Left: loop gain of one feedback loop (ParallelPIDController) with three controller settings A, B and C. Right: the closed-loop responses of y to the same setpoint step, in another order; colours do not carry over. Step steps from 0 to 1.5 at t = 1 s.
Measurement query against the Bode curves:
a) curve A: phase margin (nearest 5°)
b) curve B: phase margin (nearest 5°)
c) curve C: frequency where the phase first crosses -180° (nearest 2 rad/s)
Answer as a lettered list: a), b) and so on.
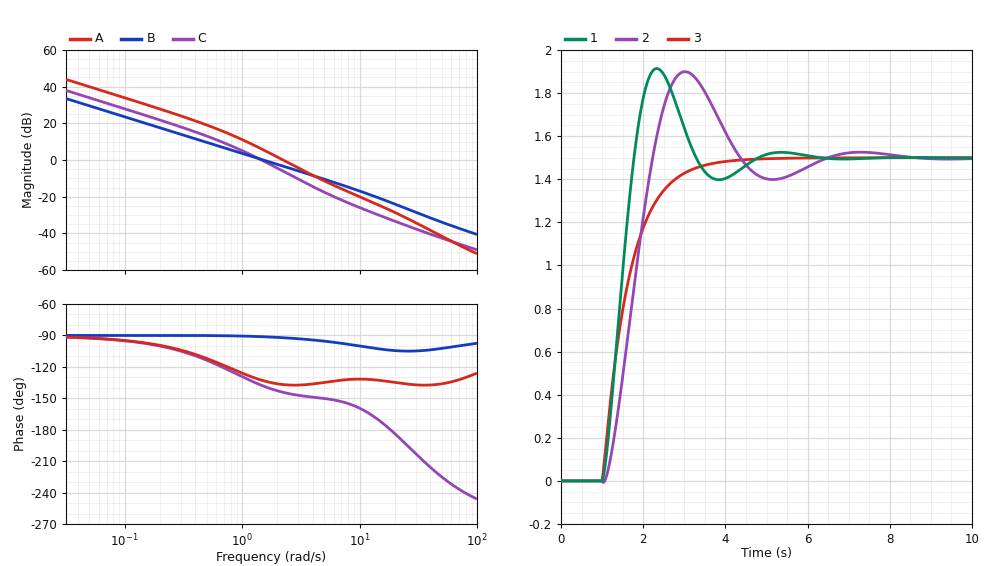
a) 45°
b) 90°
c) 18 rad/s
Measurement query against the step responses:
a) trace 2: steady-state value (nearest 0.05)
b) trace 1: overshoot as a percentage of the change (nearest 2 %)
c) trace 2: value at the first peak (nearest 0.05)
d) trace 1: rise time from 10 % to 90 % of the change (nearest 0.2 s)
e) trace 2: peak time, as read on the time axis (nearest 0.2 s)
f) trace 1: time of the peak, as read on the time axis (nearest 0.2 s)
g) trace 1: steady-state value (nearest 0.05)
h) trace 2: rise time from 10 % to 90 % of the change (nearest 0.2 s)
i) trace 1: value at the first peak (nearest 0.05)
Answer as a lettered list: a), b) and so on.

a) 1.50
b) 28 %
c) 1.90
d) 0.6 s
e) 3.0 s
f) 2.4 s
g) 1.50
h) 0.8 s
i) 1.90
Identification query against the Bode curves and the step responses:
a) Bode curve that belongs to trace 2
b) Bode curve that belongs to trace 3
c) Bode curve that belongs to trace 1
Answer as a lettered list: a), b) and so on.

a) C
b) B
c) A
